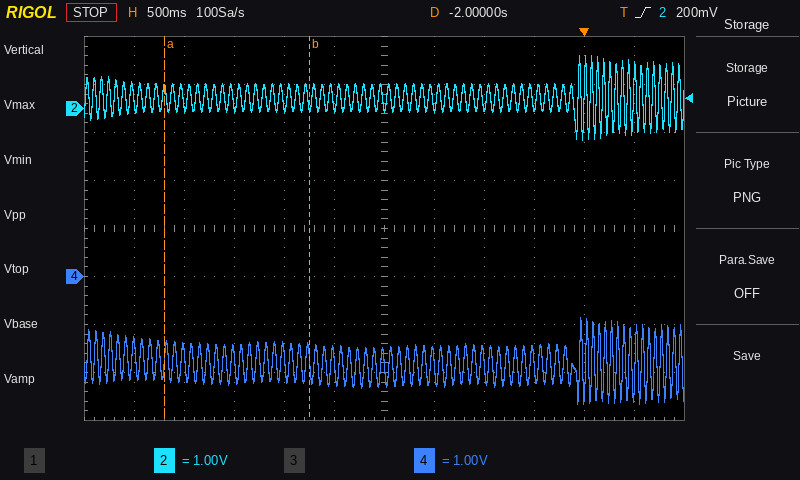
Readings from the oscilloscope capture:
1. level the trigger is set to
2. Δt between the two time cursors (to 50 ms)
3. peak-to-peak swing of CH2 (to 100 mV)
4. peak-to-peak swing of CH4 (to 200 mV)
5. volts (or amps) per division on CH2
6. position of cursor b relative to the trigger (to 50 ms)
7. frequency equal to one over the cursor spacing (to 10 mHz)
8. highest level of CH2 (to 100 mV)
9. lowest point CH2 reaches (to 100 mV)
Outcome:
200 mV
1.45 s
1.7 V
1.8 V
1 V
-2.75 s
690 mHz
1.1 V
-600 mV
